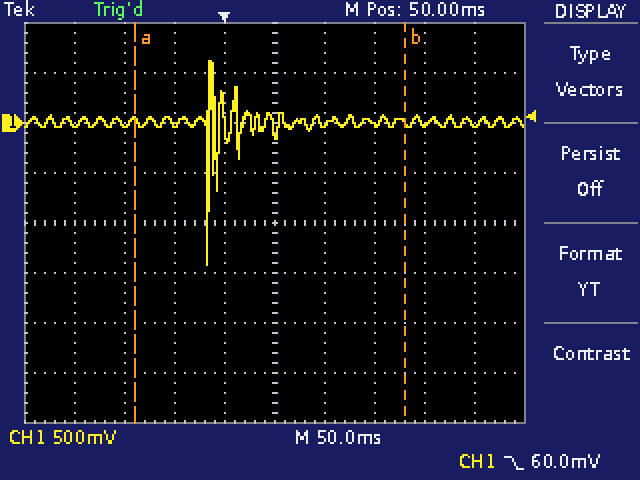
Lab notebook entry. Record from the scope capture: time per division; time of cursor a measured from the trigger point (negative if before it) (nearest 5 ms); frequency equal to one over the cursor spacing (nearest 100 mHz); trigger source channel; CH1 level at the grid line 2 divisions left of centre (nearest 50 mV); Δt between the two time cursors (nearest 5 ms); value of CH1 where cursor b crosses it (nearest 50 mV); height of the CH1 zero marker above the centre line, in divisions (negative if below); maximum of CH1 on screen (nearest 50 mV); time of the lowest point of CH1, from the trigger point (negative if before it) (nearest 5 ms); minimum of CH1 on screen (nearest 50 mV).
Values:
50 ms
-90 ms
3.7 Hz
CH1
0 mV
270 ms
0 mV
+2.0 div
600 mV
-15 ms
-1.40 V
